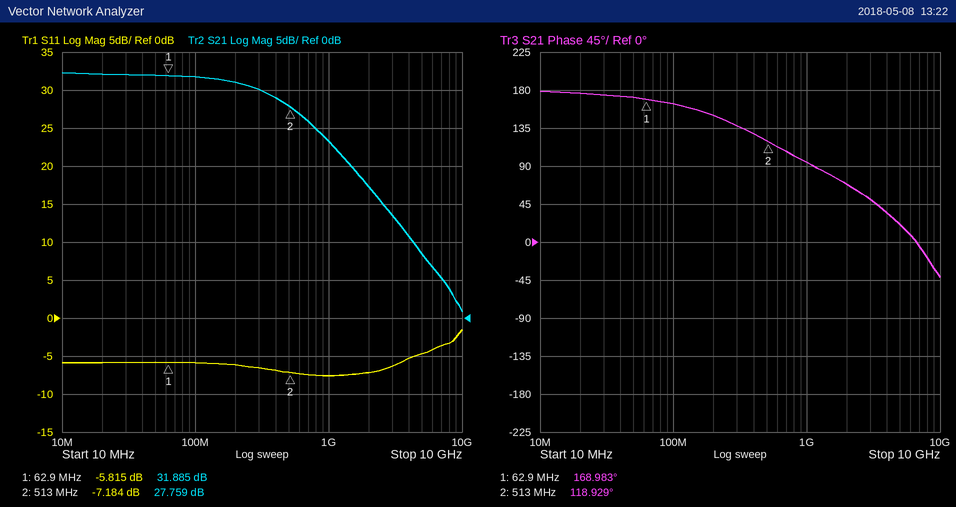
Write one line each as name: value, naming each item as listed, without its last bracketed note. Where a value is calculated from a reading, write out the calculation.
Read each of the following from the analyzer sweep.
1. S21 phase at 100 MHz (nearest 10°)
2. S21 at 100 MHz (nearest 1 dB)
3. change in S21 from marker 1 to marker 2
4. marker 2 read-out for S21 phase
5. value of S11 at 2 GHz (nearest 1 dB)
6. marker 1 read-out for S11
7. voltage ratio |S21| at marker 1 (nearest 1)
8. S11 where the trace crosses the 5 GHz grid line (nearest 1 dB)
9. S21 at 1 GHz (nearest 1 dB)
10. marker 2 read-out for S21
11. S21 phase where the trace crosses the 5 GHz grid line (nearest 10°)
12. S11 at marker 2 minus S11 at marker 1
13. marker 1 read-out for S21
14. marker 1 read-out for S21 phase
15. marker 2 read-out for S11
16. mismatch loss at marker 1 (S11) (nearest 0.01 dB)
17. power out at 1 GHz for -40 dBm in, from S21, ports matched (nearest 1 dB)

S21 phase at 100 MHz: 160°
S21 at 100 MHz: 32 dB
change in S21 from marker 1 to marker 2: 27.759 − (31.885) = -4.126 dB
marker 2 read-out for S21 phase: 118.929°
value of S11 at 2 GHz: -7 dB
marker 1 read-out for S11: -5.815 dB
voltage ratio |S21| at marker 1: 10^(31.885/20) ≈ 39
S11 where the trace crosses the 5 GHz grid line: -5 dB
S21 at 1 GHz: 23 dB
marker 2 read-out for S21: 27.759 dB
S21 phase where the trace crosses the 5 GHz grid line: 20°
S11 at marker 2 minus S11 at marker 1: -7.184 − (-5.815) = -1.369 dB
marker 1 read-out for S21: 31.885 dB
marker 1 read-out for S21 phase: 168.983°
marker 2 read-out for S11: -7.184 dB
mismatch loss at marker 1 (S11): −10 log10(1 − 10^(-5.815/10)) ≈ 1.32 dB
power out at 1 GHz for -40 dBm in, from S21, ports matched: -40 dBm + (23 dB) = -17 dBm
